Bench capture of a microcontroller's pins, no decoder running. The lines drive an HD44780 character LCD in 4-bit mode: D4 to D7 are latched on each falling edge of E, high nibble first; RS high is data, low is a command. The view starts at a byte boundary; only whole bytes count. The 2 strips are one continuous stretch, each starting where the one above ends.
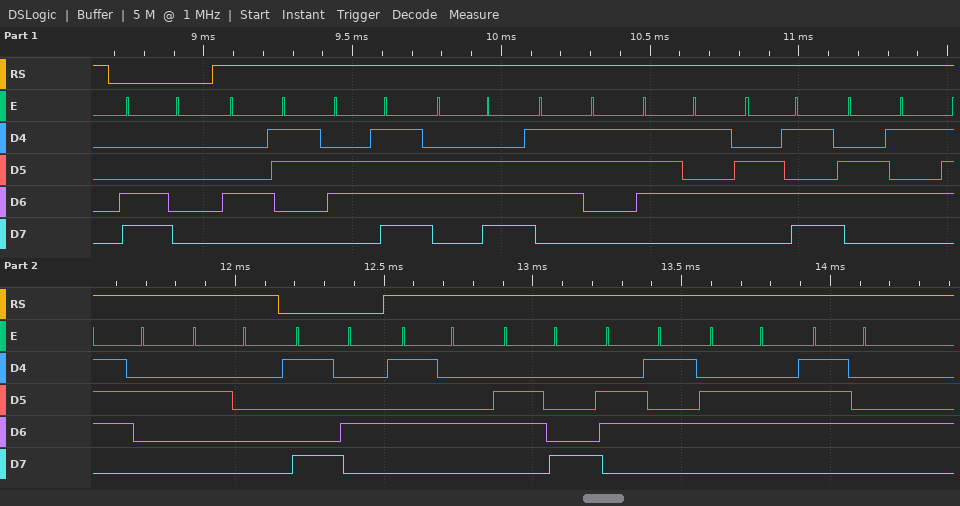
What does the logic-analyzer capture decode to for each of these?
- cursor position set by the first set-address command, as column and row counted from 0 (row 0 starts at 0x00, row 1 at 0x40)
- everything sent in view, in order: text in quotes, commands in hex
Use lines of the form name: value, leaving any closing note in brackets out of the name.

cursor position set by the first set-address command, as column and row counted from 0: column 0, row 1
everything sent in view, in order: text in quotes, commands in hex: 0xC0 "Consumer " 0x94 "Theft"
